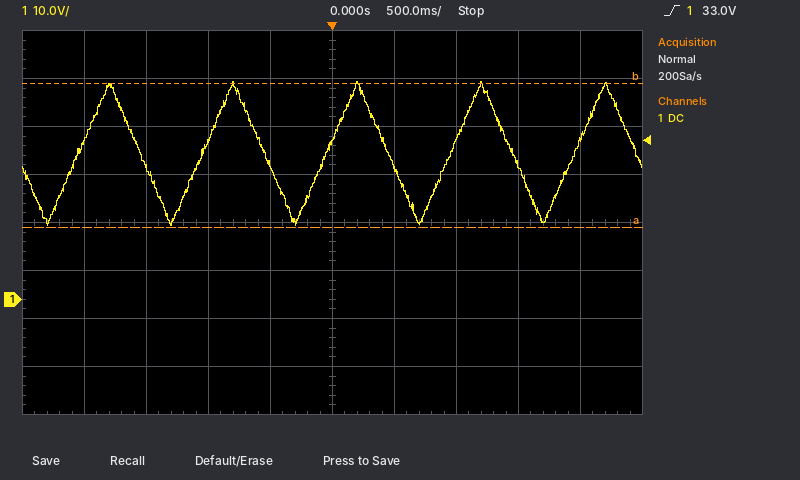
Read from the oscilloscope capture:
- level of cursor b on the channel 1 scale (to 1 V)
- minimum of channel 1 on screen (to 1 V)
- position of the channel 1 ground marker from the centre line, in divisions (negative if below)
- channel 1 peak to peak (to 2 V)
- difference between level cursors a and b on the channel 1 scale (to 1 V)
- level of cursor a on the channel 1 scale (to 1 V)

45 V
15 V
-1.6 div
30 V
30 V
15 V
